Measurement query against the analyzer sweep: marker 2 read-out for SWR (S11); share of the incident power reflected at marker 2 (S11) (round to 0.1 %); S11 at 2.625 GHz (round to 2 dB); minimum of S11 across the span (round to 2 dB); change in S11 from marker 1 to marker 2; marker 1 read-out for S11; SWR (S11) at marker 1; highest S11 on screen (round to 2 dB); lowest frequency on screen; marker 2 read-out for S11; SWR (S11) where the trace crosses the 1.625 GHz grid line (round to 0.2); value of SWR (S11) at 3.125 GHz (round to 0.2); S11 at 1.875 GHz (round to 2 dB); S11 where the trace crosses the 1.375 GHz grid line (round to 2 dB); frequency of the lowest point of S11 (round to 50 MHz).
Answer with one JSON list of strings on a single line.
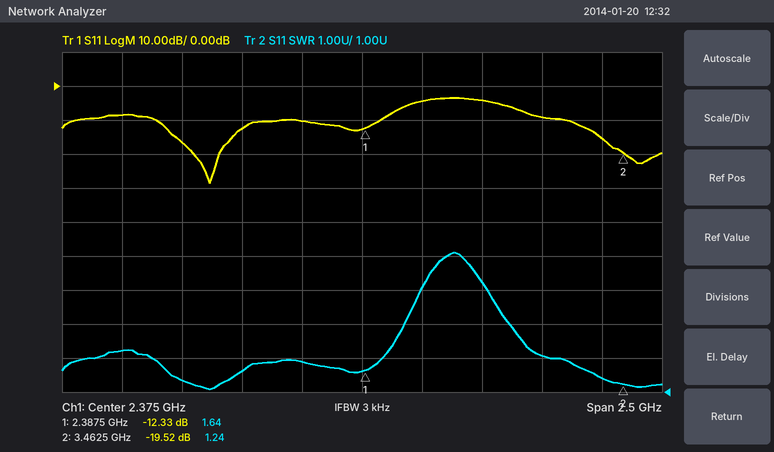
["1.24", "1.1 %", "-4 dB", "-28 dB", "-7.19 dB", "-12.33 dB", "1.64", "-4 dB", "1.125 GHz", "-19.52 dB", "1.4", "2.0", "-12 dB", "-8 dB", "1.75 GHz"]
